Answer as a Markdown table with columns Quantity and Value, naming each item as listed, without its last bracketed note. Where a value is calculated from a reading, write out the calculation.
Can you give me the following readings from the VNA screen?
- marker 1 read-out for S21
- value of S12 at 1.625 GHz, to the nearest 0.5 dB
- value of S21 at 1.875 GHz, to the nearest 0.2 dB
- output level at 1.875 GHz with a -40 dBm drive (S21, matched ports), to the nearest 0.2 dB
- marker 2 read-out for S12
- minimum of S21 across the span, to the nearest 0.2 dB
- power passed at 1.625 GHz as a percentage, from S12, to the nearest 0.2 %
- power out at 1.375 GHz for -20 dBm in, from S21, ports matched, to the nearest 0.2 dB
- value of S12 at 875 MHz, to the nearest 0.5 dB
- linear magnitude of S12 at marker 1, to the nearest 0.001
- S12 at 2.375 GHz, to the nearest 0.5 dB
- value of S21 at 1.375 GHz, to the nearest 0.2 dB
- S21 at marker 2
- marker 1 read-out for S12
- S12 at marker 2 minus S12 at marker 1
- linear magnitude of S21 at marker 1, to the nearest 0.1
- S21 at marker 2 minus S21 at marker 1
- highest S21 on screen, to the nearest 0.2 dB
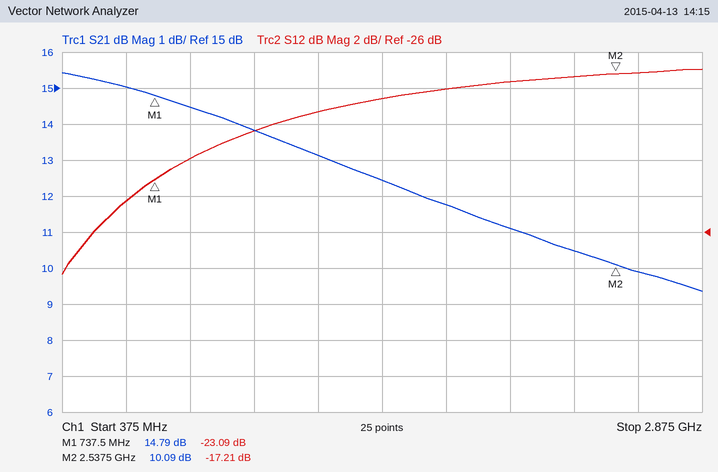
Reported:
| Quantity | Value |
|---|---|
| marker 1 read-out for S21 | 14.79 dB |
| value of S12 at 1.625 GHz, to the nearest 0.5 dB | -18.5 dB |
| value of S21 at 1.875 GHz, to the nearest 0.2 dB | 11.8 dB |
| output level at 1.875 GHz with a -40 dBm drive (S21, matched ports), to the nearest 0.2 dB | -40 dBm + (11.8 dB) = -28.2 dBm |
| marker 2 read-out for S12 | -17.21 dB |
| minimum of S21 across the span, to the nearest 0.2 dB | 9.4 dB |
| power passed at 1.625 GHz as a percentage, from S12, to the nearest 0.2 % | 10^(-18.5/10) ≈ 1.4 % |
| power out at 1.375 GHz for -20 dBm in, from S21, ports matched, to the nearest 0.2 dB | -20 dBm + (13.2 dB) = -6.8 dBm |
| value of S12 at 875 MHz, to the nearest 0.5 dB | -22.0 dB |
| linear magnitude of S12 at marker 1, to the nearest 0.001 | 10^(-23.09/20) ≈ 0.070 |
| S12 at 2.375 GHz, to the nearest 0.5 dB | -17.5 dB |
| value of S21 at 1.375 GHz, to the nearest 0.2 dB | 13.2 dB |
| S21 at marker 2 | 10.09 dB |
| marker 1 read-out for S12 | -23.09 dB |
| S12 at marker 2 minus S12 at marker 1 | -17.21 − (-23.09) = 5.88 dB |
| linear magnitude of S21 at marker 1, to the nearest 0.1 | 10^(14.79/20) ≈ 5.5 |
| S21 at marker 2 minus S21 at marker 1 | 10.09 − (14.79) = -4.70 dB |
| highest S21 on screen, to the nearest 0.2 dB | 15.4 dB |
